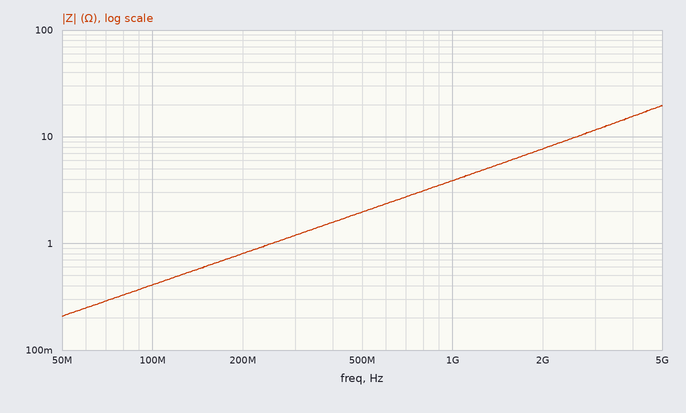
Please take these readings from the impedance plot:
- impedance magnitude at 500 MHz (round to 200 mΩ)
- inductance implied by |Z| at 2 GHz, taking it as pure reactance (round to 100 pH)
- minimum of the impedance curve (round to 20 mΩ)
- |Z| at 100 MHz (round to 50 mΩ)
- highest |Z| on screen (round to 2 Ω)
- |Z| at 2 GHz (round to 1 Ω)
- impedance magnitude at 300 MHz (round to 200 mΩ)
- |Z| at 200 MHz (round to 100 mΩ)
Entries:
2.0 Ω
600 pH
200 mΩ
400 mΩ
20 Ω
8 Ω
1.2 Ω
800 mΩ
